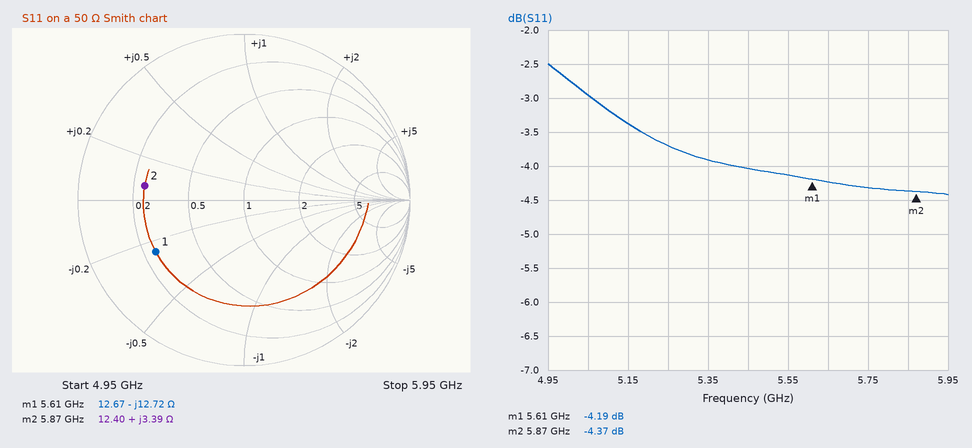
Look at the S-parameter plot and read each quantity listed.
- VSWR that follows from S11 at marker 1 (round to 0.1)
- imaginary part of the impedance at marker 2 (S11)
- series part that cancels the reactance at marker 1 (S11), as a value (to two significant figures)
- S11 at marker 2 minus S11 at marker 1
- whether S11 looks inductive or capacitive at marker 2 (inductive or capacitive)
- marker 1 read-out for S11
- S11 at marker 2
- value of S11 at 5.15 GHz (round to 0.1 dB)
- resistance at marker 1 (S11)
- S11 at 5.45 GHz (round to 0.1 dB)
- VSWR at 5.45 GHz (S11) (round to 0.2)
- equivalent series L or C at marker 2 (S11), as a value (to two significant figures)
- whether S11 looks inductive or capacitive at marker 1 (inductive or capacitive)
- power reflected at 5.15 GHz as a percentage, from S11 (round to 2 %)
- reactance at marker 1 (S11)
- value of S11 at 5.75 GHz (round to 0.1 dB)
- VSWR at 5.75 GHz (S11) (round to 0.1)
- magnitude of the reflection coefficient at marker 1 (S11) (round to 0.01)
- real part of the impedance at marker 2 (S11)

4.2
+3.39 Ω
360 pH
-0.18 dB
inductive
-4.19 dB
-4.37 dB
-3.4 dB
12.67 Ω
-4.0 dB
4.4
92 pH
capacitive
46 %
-12.72 Ω
-4.3 dB
4.1
0.62
12.40 Ω
